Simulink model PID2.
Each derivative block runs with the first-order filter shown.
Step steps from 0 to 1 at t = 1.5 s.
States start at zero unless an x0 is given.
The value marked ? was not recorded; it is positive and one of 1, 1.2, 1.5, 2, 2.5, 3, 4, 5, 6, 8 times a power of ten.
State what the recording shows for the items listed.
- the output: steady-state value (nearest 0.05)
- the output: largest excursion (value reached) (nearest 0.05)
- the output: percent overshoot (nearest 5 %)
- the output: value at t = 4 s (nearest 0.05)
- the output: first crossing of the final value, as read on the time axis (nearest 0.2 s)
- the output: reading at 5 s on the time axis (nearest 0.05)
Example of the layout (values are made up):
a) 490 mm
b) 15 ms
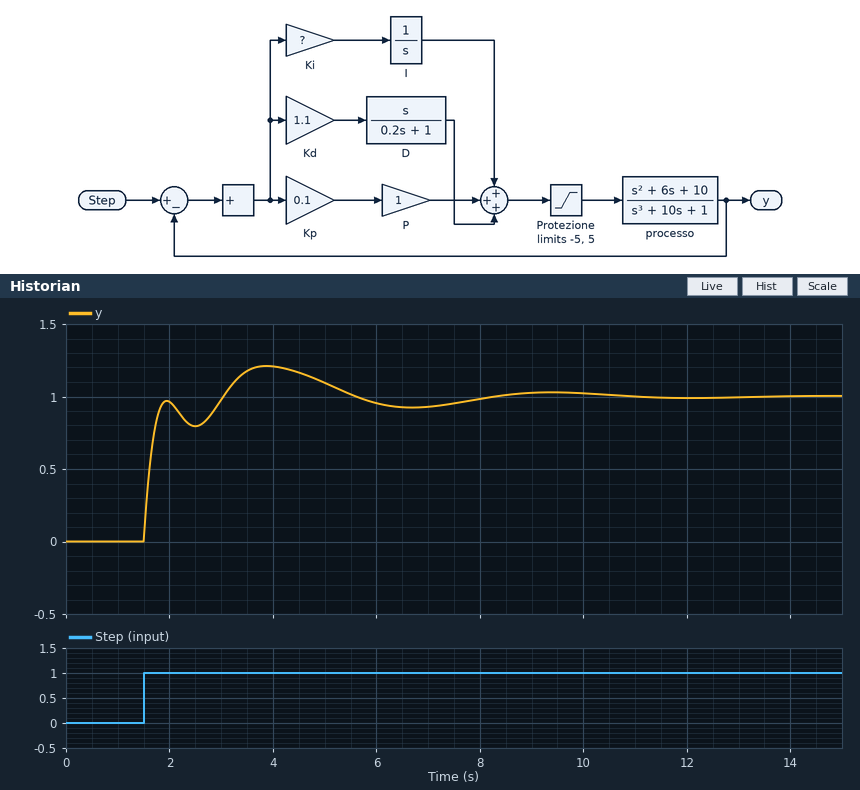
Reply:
a) 1.00
b) 1.20
c) 20 %
d) 1.20
e) 3.0 s
f) 1.10
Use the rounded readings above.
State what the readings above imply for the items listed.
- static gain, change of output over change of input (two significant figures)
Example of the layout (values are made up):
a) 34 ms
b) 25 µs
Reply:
a) 1.0
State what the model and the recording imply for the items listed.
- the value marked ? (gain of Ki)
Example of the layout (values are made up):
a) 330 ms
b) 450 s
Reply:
a) 3
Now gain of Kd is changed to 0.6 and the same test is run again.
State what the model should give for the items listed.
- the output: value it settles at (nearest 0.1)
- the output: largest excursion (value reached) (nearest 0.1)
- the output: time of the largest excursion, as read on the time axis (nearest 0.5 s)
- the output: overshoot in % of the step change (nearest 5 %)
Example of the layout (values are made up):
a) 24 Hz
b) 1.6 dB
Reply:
a) 1.0
b) 1.3
c) 3.5 s
d) 30 %
